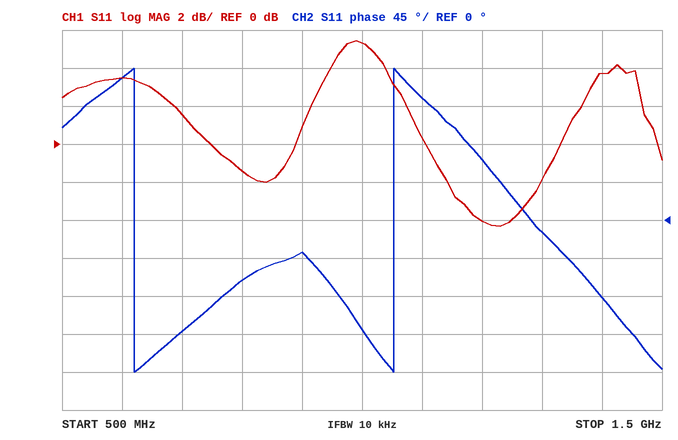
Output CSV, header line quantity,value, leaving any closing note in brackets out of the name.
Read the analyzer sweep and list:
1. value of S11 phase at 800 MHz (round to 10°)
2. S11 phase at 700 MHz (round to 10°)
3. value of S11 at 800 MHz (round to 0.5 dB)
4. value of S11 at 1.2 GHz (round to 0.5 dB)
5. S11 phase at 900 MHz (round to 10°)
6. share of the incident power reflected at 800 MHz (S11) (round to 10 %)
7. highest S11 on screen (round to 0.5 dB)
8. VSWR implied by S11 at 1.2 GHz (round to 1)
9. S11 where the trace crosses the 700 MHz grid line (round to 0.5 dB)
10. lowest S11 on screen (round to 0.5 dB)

quantity,value
value of S11 phase at 800 MHz,-70°
S11 phase at 700 MHz,-130°
value of S11 at 800 MHz,-1.5 dB
value of S11 at 1.2 GHz,-4.0 dB
S11 phase at 900 MHz,-40°
share of the incident power reflected at 800 MHz (S11),70 %
highest S11 on screen,5.5 dB
VSWR implied by S11 at 1.2 GHz,4
S11 where the trace crosses the 700 MHz grid line,1.5 dB
lowest S11 on screen,-4.5 dB
